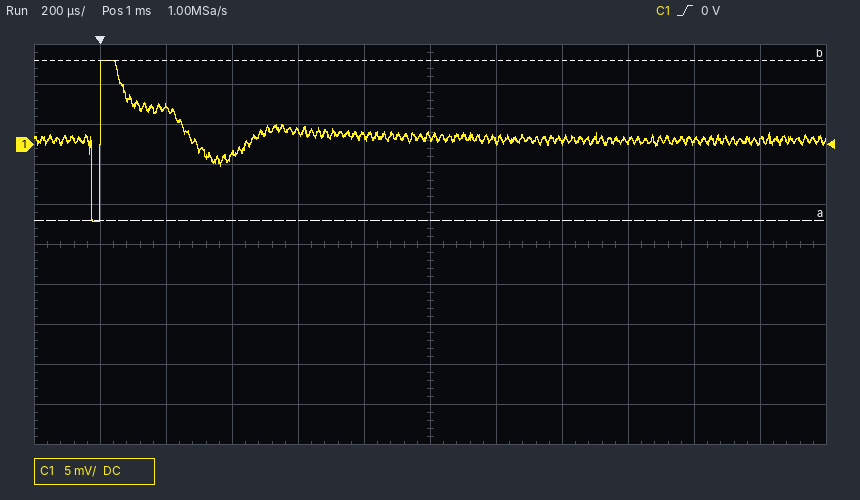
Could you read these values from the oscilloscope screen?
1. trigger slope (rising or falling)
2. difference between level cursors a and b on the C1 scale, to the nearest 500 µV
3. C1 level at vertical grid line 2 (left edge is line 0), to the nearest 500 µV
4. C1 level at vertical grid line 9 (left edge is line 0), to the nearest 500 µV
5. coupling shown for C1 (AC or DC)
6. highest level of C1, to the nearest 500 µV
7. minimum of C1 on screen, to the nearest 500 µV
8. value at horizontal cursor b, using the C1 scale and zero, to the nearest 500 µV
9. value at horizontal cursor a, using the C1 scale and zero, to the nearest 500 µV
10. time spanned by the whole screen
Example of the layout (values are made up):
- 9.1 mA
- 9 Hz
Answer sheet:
- rising
- 20.0 mV
- 4.5 mV
- 500 µV
- DC
- 10.5 mV
- -9.5 mV
- 10.5 mV
- -9.5 mV
- 2.4 ms
